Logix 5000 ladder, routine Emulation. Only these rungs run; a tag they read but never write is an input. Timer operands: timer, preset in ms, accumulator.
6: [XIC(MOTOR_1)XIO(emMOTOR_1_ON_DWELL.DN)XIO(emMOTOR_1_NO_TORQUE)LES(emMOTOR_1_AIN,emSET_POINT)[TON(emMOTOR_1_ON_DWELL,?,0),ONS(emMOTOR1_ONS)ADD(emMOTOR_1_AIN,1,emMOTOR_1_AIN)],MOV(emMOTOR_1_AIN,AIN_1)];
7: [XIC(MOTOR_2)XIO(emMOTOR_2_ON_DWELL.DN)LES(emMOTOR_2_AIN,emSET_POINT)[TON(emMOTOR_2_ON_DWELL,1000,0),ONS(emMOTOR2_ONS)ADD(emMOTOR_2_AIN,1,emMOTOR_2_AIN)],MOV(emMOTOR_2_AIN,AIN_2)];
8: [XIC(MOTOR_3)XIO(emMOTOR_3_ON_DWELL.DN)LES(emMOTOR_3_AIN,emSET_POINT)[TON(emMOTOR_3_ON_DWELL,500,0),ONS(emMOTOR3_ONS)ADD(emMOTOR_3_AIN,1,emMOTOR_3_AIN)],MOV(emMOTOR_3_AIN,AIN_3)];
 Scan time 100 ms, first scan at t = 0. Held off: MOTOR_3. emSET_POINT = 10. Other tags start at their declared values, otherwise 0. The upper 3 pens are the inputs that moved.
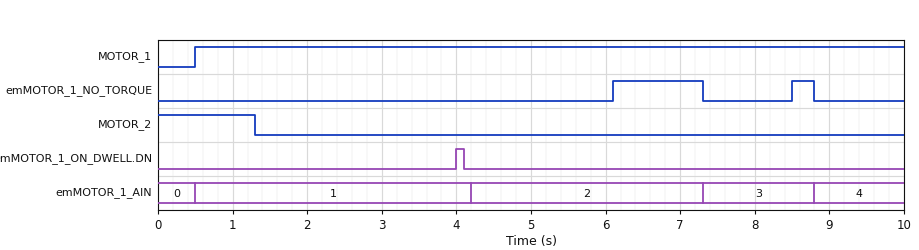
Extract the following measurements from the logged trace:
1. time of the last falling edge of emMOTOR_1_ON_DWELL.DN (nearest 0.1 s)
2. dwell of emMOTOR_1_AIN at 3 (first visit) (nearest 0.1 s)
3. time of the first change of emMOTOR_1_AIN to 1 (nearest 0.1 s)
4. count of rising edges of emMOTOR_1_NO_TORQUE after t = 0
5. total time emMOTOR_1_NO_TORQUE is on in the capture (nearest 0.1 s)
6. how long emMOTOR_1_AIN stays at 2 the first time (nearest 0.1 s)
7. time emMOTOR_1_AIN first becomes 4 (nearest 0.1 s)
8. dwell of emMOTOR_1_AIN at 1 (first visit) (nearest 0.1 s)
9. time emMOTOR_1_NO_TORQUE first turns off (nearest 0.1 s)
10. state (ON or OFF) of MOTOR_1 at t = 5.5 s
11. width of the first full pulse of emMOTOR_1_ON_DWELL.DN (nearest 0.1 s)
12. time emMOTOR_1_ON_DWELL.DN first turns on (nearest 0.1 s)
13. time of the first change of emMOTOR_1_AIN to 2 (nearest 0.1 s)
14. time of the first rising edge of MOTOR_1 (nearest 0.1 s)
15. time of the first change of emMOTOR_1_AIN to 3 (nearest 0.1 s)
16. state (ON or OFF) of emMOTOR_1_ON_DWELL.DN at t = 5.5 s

4.1 s
1.5 s
0.5 s
2
1.5 s
3.1 s
8.8 s
3.7 s
7.3 s
ON
0.1 s
4.0 s
4.2 s
0.5 s
7.3 s
OFF
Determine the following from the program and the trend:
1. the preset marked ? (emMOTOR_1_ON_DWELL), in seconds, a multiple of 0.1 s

3.5 s
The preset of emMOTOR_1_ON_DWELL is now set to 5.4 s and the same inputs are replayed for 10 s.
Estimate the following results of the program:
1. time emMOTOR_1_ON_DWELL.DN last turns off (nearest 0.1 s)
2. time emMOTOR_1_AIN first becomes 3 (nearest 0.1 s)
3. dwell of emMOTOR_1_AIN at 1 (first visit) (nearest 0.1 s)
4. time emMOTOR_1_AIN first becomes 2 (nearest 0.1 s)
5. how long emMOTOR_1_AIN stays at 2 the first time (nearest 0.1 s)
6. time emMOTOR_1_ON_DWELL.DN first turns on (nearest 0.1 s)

6.0 s
8.8 s
6.8 s
7.3 s
1.5 s
5.9 s
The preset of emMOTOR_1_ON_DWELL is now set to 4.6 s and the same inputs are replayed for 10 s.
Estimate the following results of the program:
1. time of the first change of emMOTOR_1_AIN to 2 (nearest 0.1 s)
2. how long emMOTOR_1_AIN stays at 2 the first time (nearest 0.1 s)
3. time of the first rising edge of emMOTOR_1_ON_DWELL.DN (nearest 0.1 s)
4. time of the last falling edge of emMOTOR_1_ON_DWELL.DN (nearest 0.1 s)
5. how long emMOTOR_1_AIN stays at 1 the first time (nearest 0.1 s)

5.3 s
2.0 s
5.1 s
5.2 s
4.8 s
